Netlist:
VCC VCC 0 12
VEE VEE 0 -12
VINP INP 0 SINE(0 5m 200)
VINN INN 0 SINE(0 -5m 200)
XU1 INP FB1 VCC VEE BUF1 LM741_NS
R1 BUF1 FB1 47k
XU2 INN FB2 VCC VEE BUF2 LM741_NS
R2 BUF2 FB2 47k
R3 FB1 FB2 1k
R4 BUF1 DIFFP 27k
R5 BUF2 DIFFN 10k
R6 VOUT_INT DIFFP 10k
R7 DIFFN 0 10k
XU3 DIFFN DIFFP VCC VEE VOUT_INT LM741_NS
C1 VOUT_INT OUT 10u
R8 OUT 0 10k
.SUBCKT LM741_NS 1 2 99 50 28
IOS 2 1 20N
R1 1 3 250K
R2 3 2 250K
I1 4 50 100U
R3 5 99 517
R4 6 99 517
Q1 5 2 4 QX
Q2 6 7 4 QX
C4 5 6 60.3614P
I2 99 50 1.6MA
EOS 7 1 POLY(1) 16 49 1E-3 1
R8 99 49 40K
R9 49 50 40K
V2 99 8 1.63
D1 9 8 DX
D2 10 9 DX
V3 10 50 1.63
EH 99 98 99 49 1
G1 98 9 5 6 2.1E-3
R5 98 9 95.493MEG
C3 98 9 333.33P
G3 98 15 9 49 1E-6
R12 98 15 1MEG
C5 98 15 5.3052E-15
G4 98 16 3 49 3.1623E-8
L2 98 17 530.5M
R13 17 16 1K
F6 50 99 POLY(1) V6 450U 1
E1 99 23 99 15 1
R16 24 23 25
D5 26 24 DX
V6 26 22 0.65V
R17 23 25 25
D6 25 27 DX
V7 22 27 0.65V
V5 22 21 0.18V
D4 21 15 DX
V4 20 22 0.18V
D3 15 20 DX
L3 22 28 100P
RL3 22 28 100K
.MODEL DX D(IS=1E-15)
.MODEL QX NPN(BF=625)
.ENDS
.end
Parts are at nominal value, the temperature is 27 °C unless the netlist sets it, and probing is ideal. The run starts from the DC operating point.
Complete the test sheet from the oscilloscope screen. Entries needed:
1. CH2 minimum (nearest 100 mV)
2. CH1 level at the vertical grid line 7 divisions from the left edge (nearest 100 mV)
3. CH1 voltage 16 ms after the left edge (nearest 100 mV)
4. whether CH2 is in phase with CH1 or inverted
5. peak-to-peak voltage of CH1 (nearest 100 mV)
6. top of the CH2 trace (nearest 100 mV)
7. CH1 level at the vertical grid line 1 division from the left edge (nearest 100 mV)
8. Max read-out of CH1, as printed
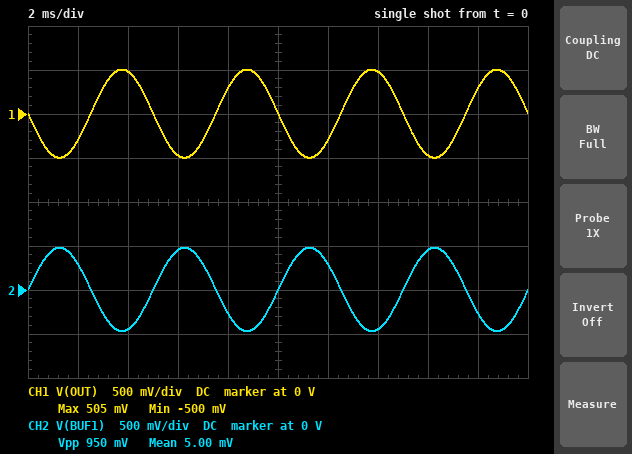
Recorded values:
-500 mV
500 mV
-500 mV
inverted
1.0 V
500 mV
-300 mV
505 mV
